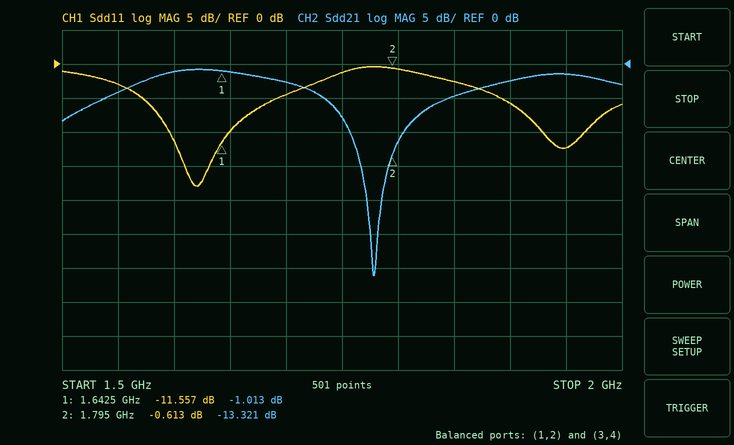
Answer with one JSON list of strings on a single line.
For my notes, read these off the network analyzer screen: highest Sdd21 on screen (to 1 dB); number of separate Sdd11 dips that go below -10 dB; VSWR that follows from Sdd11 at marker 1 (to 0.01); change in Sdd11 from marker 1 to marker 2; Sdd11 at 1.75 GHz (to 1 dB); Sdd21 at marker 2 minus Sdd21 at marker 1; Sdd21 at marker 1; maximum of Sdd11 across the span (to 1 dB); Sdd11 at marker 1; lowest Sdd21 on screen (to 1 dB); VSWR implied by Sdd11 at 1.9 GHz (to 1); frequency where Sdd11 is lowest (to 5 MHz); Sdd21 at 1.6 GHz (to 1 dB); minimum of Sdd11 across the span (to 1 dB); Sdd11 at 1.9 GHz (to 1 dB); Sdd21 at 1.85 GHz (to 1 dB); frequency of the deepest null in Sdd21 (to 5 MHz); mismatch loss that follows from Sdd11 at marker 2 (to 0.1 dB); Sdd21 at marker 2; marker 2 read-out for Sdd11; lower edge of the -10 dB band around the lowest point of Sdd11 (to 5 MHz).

["-1 dB", "2", "1.72", "10.944 dB", "-1 dB", "-12.308 dB", "-1.013 dB", "0 dB", "-11.557 dB", "-31 dB", "3", "1.620 GHz", "-1 dB", "-18 dB", "-6 dB", "-5 dB", "1.780 GHz", "8.8 dB", "-13.321 dB", "-0.613 dB", "1.595 GHz"]
